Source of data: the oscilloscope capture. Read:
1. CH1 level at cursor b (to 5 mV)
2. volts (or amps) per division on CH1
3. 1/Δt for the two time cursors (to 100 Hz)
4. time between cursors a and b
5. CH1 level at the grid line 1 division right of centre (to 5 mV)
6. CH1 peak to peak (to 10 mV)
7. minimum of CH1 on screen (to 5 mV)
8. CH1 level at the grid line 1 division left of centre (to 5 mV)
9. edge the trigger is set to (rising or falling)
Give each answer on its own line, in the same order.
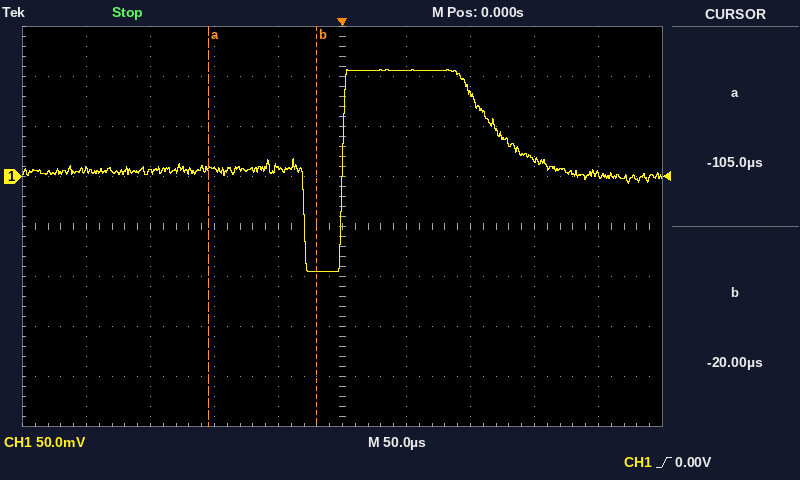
-95 mV
50 mV
11.8 kHz
85 µs
105 mV
200 mV
-95 mV
10 mV
rising
